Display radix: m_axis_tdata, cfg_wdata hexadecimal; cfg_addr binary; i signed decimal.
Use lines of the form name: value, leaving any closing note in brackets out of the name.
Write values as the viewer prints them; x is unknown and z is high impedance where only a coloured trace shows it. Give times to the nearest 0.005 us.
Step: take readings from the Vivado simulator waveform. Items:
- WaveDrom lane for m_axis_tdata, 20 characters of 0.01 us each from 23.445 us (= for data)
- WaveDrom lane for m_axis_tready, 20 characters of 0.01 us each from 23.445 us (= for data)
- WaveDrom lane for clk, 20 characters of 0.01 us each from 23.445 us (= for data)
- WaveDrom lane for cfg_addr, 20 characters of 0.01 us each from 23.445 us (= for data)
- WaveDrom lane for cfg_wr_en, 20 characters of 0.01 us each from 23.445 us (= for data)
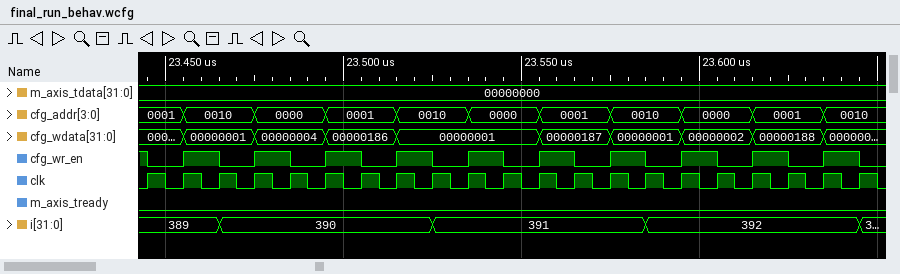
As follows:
WaveDrom lane for m_axis_tdata, 20 characters of 0.01 us each from 23.445 us: {name: 'm_axis_tdata', wave: '=...................', data: '00000000'}
WaveDrom lane for m_axis_tready, 20 characters of 0.01 us each from 23.445 us: {name: 'm_axis_tready', wave: '0...................'}
WaveDrom lane for clk, 20 characters of 0.01 us each from 23.445 us: {name: 'clk', wave: 'p...................'}
WaveDrom lane for cfg_addr, 20 characters of 0.01 us each from 23.445 us: {name: 'cfg_addr', wave: '==.=.=.=.=.=.=.=.=.=', data: '0001 0010 0000 0001 0010 0000 0001 0010 0000 0001 0010'}
WaveDrom lane for cfg_wr_en, 20 characters of 0.01 us each from 23.445 us: {name: 'cfg_wr_en', wave: '01010101010101010101'}
